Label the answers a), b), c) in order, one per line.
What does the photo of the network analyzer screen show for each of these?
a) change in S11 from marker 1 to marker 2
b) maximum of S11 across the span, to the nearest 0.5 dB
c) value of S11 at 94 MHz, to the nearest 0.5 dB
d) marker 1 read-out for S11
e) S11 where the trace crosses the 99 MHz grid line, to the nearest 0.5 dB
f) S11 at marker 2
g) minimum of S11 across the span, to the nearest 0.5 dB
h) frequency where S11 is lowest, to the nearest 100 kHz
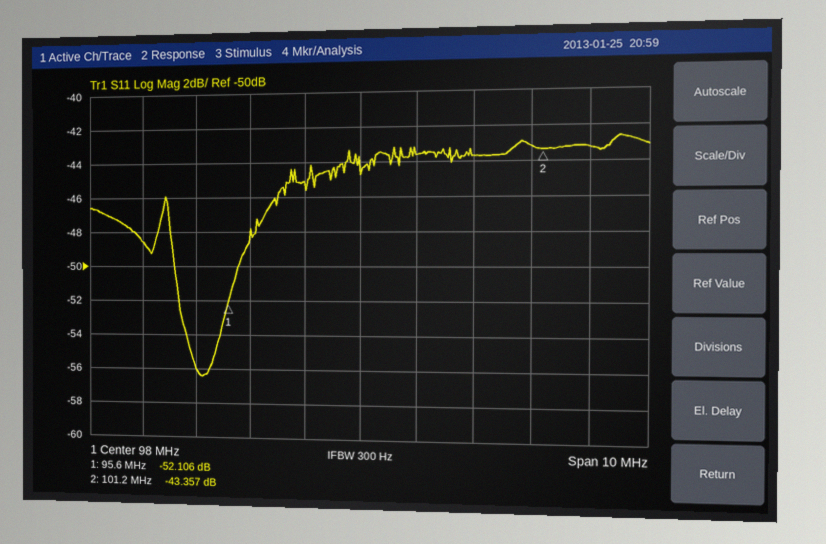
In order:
a) 8.749 dB
b) -42.5 dB
c) -48.5 dB
d) -52.106 dB
e) -43.5 dB
f) -43.357 dB
g) -56.5 dB
h) 95.1 MHz
